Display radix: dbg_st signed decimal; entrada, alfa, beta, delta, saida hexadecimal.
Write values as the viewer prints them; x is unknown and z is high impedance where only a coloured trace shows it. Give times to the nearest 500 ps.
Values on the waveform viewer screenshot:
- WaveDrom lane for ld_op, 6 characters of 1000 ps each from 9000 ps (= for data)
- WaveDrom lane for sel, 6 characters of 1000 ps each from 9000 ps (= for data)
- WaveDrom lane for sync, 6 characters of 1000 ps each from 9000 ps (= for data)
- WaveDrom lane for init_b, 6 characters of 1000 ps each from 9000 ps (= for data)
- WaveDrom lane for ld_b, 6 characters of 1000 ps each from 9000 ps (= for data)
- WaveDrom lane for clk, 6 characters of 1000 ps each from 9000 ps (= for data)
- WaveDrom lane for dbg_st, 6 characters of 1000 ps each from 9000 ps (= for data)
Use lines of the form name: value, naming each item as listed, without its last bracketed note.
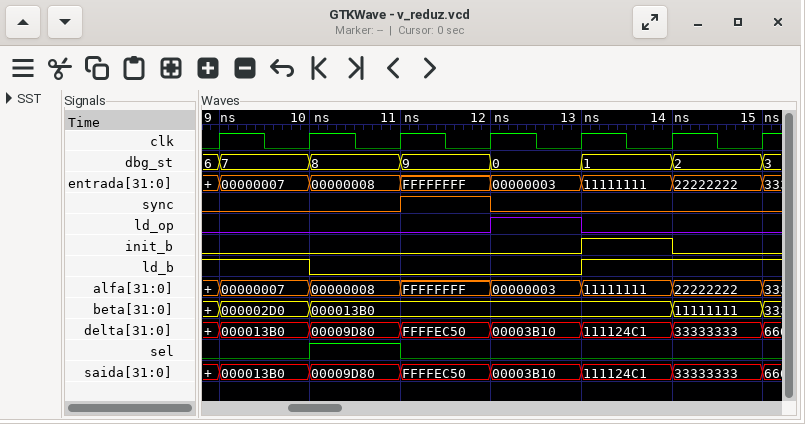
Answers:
WaveDrom lane for ld_op, 6 characters of 1000 ps each from 9000 ps: {name: 'ld_op', wave: '0..10.'}
WaveDrom lane for sel, 6 characters of 1000 ps each from 9000 ps: {name: 'sel', wave: '010...'}
WaveDrom lane for sync, 6 characters of 1000 ps each from 9000 ps: {name: 'sync', wave: '0.10..'}
WaveDrom lane for init_b, 6 characters of 1000 ps each from 9000 ps: {name: 'init_b', wave: '0...10'}
WaveDrom lane for ld_b, 6 characters of 1000 ps each from 9000 ps: {name: 'ld_b', wave: '10..1.'}
WaveDrom lane for clk, 6 characters of 1000 ps each from 9000 ps: {name: 'clk', wave: 'p.....'}
WaveDrom lane for dbg_st, 6 characters of 1000 ps each from 9000 ps: {name: 'dbg_st', wave: '======', data: '7 8 9 0 1 2'}
